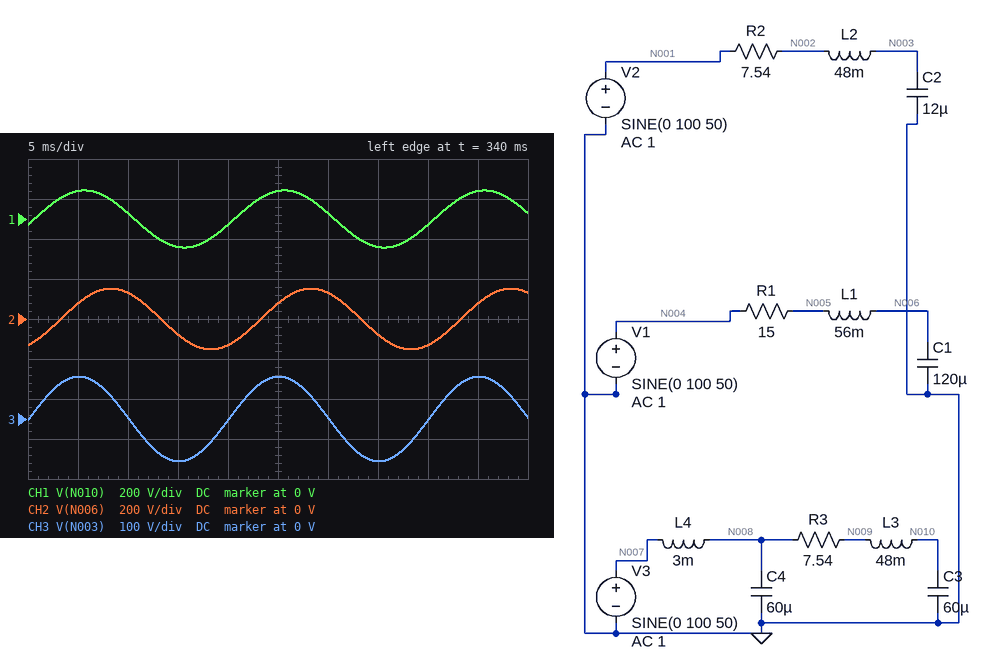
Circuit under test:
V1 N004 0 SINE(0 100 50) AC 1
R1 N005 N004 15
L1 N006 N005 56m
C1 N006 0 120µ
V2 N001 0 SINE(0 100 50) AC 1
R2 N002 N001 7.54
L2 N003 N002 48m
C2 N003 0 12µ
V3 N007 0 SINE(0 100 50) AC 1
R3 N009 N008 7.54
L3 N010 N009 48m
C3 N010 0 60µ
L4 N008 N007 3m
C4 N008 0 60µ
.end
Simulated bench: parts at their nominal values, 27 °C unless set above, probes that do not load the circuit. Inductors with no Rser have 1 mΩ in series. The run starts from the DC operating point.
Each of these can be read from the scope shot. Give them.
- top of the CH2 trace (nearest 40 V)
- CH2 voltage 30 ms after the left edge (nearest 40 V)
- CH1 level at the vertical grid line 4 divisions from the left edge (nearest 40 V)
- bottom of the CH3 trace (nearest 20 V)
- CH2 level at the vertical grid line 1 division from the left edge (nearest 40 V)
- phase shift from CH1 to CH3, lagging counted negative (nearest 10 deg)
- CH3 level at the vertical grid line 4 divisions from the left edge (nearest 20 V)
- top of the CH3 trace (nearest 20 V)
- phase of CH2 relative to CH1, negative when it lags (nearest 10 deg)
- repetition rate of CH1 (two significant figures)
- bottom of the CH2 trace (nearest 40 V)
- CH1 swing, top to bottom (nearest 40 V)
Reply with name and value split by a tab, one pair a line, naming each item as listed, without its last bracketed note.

top of the CH2 trace	160 V
CH2 voltage 30 ms after the left edge	120 V
CH1 level at the vertical grid line 4 divisions from the left edge	-40 V
bottom of the CH3 trace	-100 V
CH2 level at the vertical grid line 1 division from the left edge	80 V
phase shift from CH1 to CH3, lagging counted negative	10 deg
CH3 level at the vertical grid line 4 divisions from the left edge	0 V
top of the CH3 trace	100 V
phase of CH2 relative to CH1, negative when it lags	-50 deg
repetition rate of CH1	50 Hz
bottom of the CH2 trace	-160 V
CH1 swing, top to bottom	280 V
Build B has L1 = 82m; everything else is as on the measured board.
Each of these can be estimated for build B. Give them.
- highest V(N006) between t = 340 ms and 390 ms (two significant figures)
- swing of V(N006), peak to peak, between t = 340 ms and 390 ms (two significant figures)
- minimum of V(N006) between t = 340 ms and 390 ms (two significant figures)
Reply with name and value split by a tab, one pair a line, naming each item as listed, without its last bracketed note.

highest V(N006) between t = 340 ms and 390 ms	180 V
swing of V(N006), peak to peak, between t = 340 ms and 390 ms	350 V
minimum of V(N006) between t = 340 ms and 390 ms	-180 V
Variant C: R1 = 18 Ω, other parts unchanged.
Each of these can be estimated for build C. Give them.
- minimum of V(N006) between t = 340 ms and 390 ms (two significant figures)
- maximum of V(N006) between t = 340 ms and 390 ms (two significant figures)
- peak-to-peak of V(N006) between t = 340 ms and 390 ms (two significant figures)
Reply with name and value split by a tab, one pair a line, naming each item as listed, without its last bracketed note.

minimum of V(N006) between t = 340 ms and 390 ms	-130 V
maximum of V(N006) between t = 340 ms and 390 ms	130 V
peak-to-peak of V(N006) between t = 340 ms and 390 ms	260 V
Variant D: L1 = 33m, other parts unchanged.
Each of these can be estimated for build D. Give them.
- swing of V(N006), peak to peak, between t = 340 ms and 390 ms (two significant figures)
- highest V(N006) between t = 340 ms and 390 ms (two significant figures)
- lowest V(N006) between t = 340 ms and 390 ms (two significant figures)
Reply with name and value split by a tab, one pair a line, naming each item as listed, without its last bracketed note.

swing of V(N006), peak to peak, between t = 340 ms and 390 ms	240 V
highest V(N006) between t = 340 ms and 390 ms	120 V
lowest V(N006) between t = 340 ms and 390 ms	-120 V
